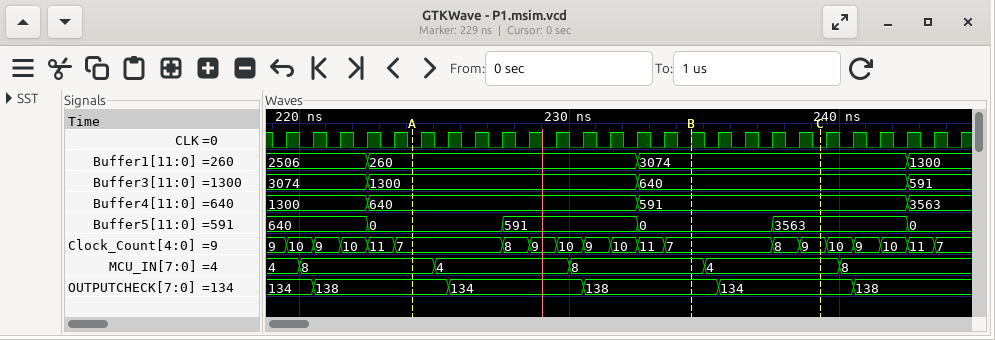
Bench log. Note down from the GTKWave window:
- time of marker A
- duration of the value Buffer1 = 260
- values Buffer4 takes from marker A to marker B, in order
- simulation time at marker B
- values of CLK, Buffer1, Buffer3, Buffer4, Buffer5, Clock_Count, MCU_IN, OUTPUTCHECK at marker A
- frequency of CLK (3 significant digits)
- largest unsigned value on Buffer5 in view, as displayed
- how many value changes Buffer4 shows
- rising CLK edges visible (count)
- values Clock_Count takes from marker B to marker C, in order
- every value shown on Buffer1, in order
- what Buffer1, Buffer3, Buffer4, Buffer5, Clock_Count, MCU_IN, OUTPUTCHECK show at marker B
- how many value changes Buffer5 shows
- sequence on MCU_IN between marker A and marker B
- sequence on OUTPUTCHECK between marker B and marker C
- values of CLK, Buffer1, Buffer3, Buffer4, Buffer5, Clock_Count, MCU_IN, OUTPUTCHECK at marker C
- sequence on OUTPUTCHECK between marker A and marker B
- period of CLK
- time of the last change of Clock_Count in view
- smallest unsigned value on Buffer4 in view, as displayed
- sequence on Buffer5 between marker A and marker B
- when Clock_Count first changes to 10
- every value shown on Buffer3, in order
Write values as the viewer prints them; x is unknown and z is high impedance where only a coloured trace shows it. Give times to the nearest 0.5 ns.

224 ns
10 ns
640, 591
234.5 ns
CLK=0, Buffer1=260, Buffer3=1300, Buffer4=640, Buffer5=0, Clock_Count=7, MCU_IN=8, OUTPUTCHECK=138
1.00 GHz
3563
3
26
7, 8, 9
2506, 260, 3074, 1300
Buffer1=3074, Buffer3=640, Buffer4=591, Buffer5=0, Clock_Count=7, MCU_IN=8, OUTPUTCHECK=138
5
8, 4, 8
138, 134
CLK=0, Buffer1=3074, Buffer3=640, Buffer4=591, Buffer5=3563, Clock_Count=9, MCU_IN=4, OUTPUTCHECK=134
138, 134, 138
1 ns
243.5 ns
591
0, 591, 0
219.5 ns
3074, 1300, 640, 591
